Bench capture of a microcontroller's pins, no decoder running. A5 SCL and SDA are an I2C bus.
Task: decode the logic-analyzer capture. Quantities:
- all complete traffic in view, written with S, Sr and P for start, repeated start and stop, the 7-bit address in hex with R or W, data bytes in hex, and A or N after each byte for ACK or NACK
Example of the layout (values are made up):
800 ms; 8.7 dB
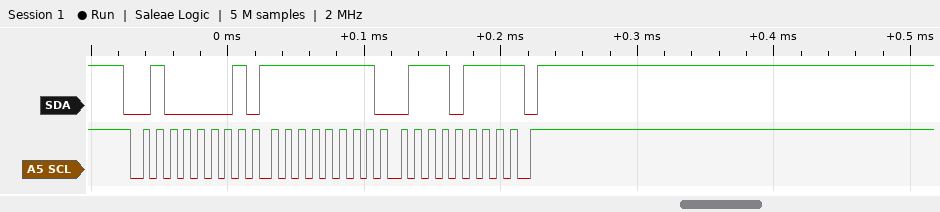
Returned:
S 20R A FF A 77 N P
